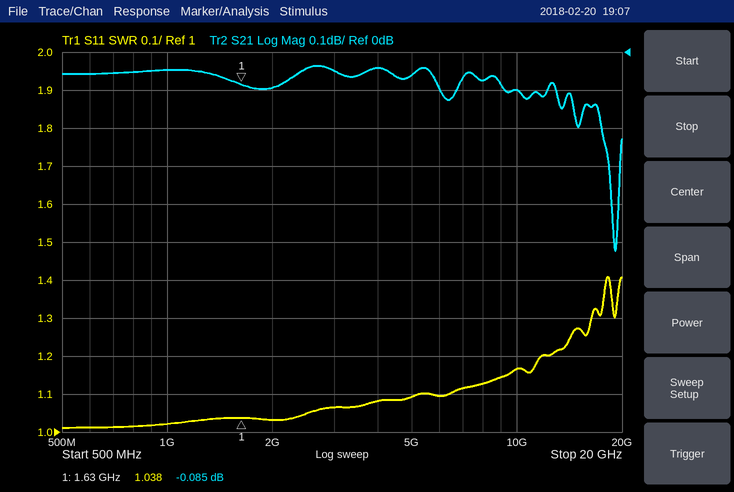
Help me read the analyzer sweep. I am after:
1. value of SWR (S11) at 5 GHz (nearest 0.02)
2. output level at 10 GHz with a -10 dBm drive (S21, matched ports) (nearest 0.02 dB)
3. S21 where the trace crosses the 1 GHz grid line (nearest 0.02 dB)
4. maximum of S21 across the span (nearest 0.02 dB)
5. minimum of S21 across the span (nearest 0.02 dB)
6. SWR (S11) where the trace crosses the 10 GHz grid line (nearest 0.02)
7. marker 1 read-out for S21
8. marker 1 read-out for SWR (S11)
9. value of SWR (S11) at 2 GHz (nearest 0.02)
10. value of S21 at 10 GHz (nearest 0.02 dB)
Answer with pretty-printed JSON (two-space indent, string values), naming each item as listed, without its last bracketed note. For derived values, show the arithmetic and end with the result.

{
  "value of SWR (S11) at 5 GHz": "1.10",
  "output level at 10 GHz with a -10 dBm drive (S21, matched ports)": "-10 dBm + (-0.10 dB) = -10.10 dBm",
  "S21 where the trace crosses the 1 GHz grid line": "-0.04 dB",
  "maximum of S21 across the span": "-0.04 dB",
  "minimum of S21 across the span": "-0.52 dB",
  "SWR (S11) where the trace crosses the 10 GHz grid line": "1.16",
  "marker 1 read-out for S21": "-0.085 dB",
  "marker 1 read-out for SWR": "1.038",
  "value of SWR (S11) at 2 GHz": "1.04",
  "value of S21 at 10 GHz": "-0.10 dB"
}
